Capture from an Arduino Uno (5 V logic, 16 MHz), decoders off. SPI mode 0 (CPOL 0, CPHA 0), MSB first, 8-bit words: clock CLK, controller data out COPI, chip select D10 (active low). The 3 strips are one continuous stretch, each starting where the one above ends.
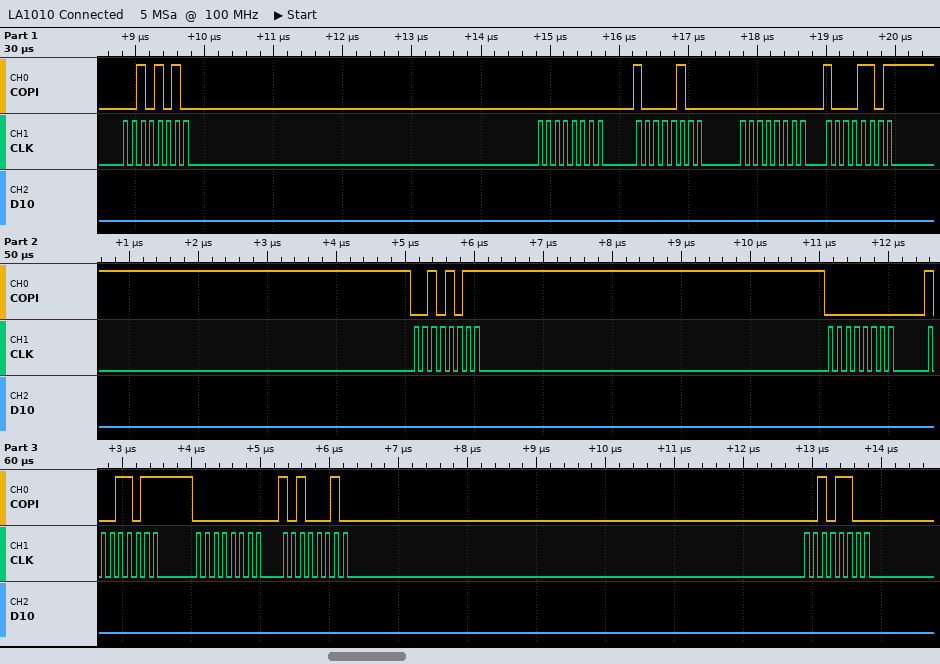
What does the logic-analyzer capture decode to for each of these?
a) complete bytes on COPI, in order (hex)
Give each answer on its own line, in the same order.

0x2A 0x00 0x84 0x00 0x8D 0x2B 0x00 0x9B 0x00 0xA2 0x2C
